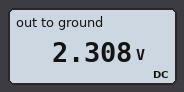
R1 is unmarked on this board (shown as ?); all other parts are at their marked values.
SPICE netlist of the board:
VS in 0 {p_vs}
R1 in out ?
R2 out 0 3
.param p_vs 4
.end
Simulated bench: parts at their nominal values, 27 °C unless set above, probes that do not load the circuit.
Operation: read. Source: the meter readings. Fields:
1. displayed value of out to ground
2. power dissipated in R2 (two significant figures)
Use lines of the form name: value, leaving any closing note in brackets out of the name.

displayed value of out to ground: 2.308 V
power dissipated in R2: 1.8 W
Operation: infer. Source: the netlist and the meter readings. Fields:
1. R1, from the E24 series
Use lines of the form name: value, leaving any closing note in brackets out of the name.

R1, from the E24 series: 2.2 Ω
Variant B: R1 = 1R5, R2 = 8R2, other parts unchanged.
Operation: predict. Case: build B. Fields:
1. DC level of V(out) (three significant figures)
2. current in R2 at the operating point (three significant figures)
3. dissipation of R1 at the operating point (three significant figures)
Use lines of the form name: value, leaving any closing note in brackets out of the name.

DC level of V(out): 3.38 V
current in R2 at the operating point: 412 mA
dissipation of R1 at the operating point: 255 mW
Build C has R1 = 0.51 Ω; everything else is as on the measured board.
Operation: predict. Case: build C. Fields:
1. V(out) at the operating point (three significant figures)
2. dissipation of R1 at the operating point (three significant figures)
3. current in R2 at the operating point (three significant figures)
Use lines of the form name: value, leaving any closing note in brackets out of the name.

V(out) at the operating point: 3.42 V
dissipation of R1 at the operating point: 662 mW
current in R2 at the operating point: 1.14 A
